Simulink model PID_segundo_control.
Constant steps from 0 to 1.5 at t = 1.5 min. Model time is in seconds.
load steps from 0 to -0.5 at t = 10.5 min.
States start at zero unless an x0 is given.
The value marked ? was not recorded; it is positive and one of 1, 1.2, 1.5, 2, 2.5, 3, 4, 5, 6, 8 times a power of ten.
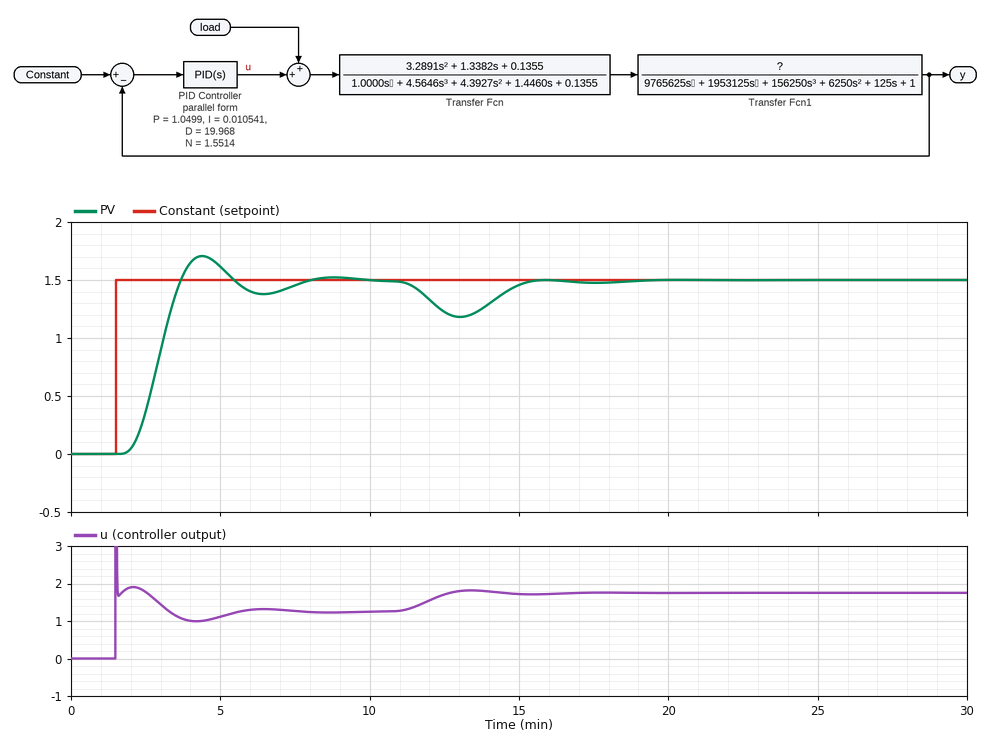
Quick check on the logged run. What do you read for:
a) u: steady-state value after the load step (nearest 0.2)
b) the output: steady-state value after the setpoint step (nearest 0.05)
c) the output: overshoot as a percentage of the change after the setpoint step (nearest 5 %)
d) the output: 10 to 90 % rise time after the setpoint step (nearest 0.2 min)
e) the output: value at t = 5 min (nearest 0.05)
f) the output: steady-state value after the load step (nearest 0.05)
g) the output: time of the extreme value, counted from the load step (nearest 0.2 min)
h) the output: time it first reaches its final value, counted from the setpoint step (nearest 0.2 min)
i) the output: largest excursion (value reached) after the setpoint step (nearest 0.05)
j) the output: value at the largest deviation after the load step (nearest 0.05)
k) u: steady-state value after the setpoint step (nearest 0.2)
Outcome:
1.8
1.50
15 %
1.2 min
1.60
1.50
2.6 min
2.2 min
1.70
1.20
1.2
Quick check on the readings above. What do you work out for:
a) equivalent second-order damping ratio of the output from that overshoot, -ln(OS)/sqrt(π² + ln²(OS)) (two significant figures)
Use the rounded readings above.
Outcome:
0.52
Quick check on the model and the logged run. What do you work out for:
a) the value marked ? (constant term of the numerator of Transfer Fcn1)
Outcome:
1.2
